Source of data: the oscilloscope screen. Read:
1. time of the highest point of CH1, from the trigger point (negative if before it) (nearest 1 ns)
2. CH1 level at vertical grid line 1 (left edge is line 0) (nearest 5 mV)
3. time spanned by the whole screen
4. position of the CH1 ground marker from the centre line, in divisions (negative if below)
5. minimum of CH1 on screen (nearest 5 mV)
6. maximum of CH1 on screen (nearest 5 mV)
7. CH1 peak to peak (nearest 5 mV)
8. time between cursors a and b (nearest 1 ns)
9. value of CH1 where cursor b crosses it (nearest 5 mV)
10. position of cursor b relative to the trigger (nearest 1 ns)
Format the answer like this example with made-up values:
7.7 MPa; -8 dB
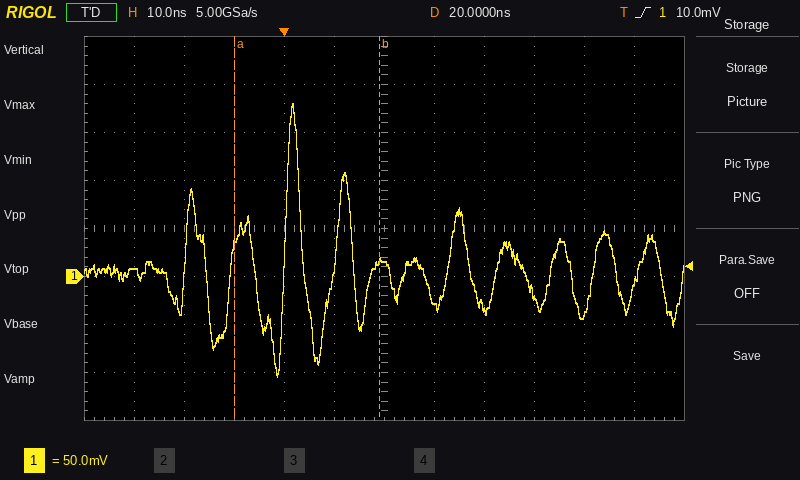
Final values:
+2 ns; 10 mV; 120 ns; -1.0 div; -105 mV; 180 mV; 285 mV; 29 ns; 15 mV; +19 ns
